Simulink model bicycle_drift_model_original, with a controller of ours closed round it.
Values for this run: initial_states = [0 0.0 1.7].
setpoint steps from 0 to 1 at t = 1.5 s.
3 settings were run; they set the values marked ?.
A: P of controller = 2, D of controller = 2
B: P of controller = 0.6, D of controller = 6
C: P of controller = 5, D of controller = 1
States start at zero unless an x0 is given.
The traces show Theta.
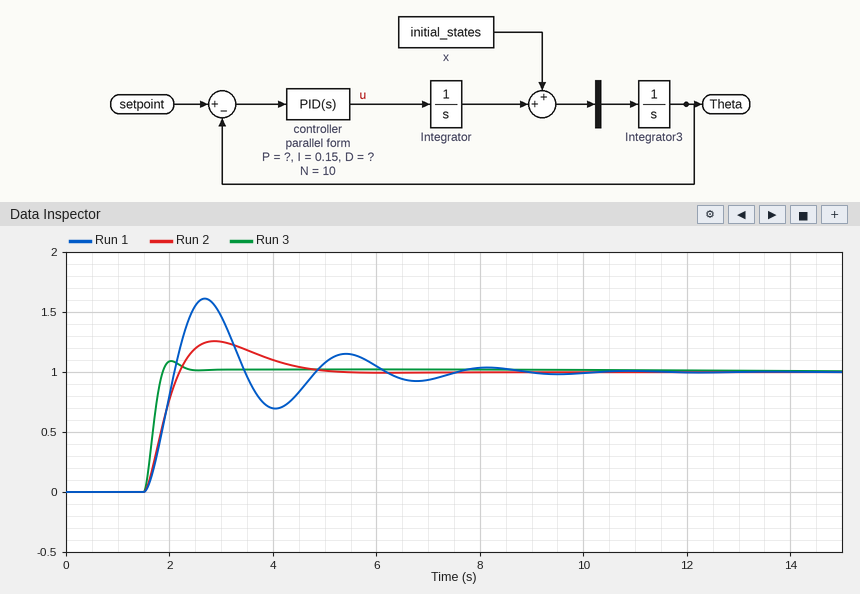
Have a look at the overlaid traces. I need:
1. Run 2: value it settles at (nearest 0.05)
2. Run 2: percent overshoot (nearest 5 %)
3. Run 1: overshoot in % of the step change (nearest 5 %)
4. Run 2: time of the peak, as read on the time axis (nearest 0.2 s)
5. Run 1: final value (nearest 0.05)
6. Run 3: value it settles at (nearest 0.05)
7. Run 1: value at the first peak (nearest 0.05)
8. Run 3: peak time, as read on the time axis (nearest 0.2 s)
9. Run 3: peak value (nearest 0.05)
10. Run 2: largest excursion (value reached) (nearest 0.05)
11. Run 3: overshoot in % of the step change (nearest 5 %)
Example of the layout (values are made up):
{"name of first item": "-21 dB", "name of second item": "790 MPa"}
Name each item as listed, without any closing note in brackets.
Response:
{"Run 2: value it settles at": "1.00", "Run 2: percent overshoot": "25 %", "Run 1: overshoot in % of the step change": "60 %", "Run 2: time of the peak, as read on the time axis": "2.8 s", "Run 1: final value": "1.00", "Run 3: value it settles at": "1.00", "Run 1: value at the first peak": "1.60", "Run 3: peak time, as read on the time axis": "2.0 s", "Run 3: peak value": "1.10", "Run 2: largest excursion (value reached)": "1.25", "Run 3: overshoot in % of the step change": "10 %"}
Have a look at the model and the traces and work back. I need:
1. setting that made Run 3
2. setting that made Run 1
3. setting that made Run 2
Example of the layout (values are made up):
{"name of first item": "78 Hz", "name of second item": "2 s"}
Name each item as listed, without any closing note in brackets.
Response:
{"setting that made Run 3": "B", "setting that made Run 1": "C", "setting that made Run 2": "A"}
